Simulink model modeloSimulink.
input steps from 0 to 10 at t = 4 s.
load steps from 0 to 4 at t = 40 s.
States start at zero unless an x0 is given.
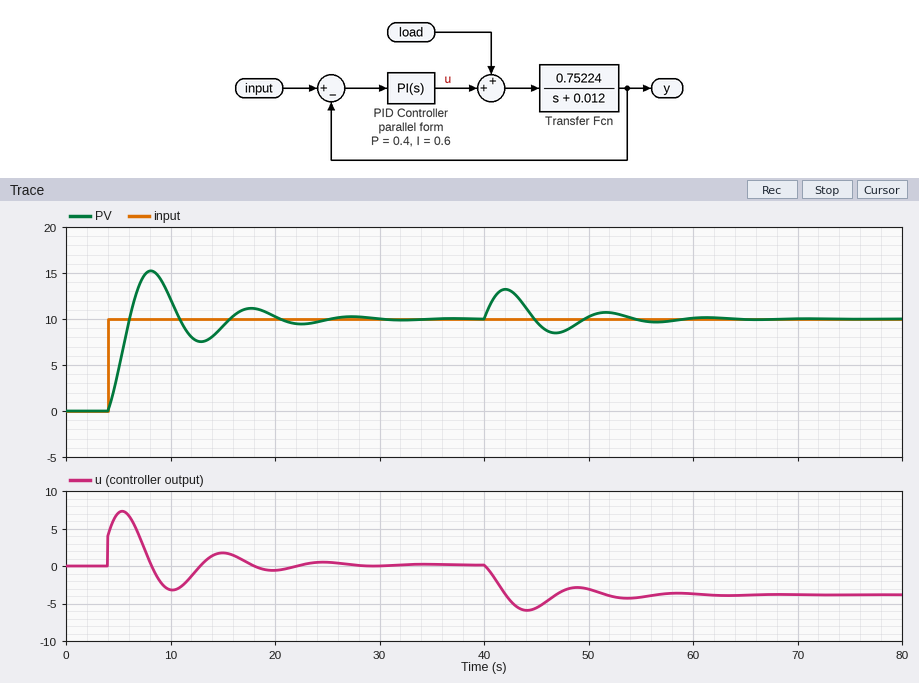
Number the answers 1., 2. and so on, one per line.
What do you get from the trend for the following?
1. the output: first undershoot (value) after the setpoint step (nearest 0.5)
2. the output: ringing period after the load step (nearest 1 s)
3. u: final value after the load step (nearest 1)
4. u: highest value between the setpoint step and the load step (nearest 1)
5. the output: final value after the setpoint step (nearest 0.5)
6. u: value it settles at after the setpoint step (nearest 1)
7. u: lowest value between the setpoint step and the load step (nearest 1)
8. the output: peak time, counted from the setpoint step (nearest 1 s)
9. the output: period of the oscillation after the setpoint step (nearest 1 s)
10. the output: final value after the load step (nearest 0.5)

1. 7.5
2. 10 s
3. -4
4. 7
5. 10.0
6. 0
7. -3
8. 4 s
9. 10 s
10. 10.0
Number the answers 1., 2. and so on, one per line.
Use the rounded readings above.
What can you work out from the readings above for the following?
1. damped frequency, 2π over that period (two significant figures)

1. 0.63 rad/s
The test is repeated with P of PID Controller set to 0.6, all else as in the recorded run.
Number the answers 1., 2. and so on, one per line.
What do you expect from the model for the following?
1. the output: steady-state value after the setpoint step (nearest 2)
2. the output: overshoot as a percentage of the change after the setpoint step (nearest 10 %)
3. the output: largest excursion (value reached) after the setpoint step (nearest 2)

1. 10
2. 40 %
3. 14
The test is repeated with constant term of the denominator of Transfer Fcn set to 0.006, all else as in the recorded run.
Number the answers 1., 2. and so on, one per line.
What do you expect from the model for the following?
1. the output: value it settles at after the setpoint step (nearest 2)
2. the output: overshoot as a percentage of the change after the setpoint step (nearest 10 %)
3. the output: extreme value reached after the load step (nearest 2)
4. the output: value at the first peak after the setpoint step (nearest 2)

1. 10
2. 50 %
3. 14
4. 16
